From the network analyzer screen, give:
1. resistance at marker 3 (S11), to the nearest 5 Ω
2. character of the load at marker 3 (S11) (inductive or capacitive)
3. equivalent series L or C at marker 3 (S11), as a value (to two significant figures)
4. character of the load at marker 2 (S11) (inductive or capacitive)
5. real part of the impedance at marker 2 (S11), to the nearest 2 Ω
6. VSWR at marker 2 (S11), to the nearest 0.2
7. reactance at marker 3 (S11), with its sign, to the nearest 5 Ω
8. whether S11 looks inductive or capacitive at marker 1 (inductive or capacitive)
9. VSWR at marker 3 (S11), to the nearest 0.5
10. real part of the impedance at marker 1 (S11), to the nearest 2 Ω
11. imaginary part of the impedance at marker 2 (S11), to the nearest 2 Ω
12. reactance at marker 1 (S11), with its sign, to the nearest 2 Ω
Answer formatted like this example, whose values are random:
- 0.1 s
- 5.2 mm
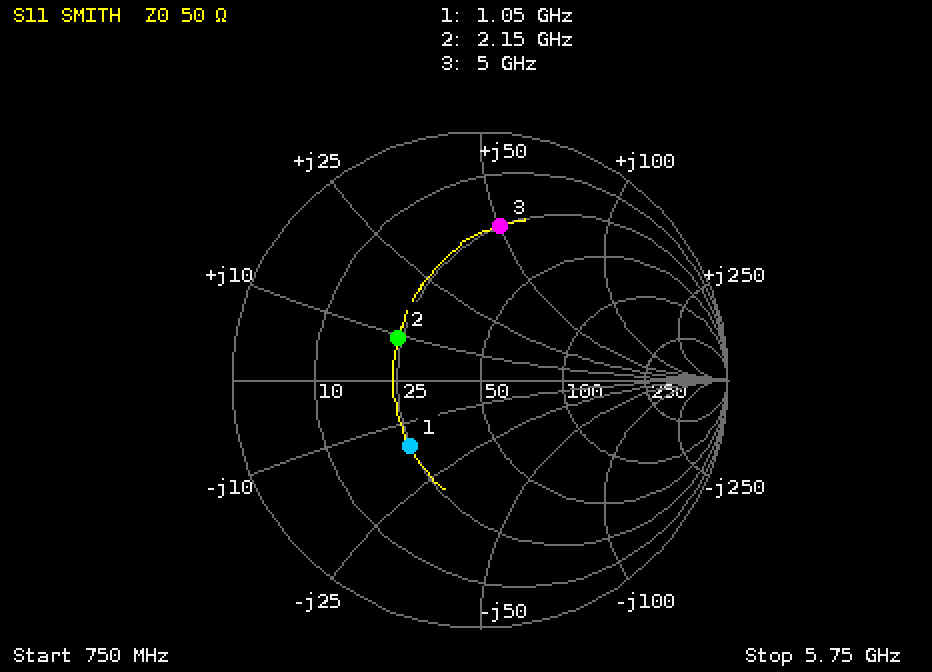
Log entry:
- 25 Ω
- inductive
- 1.6 nH
- inductive
- 24 Ω
- 2.2
- +50 Ω
- capacitive
- 4.5
- 24 Ω
- +10 Ω
- -16 Ω
